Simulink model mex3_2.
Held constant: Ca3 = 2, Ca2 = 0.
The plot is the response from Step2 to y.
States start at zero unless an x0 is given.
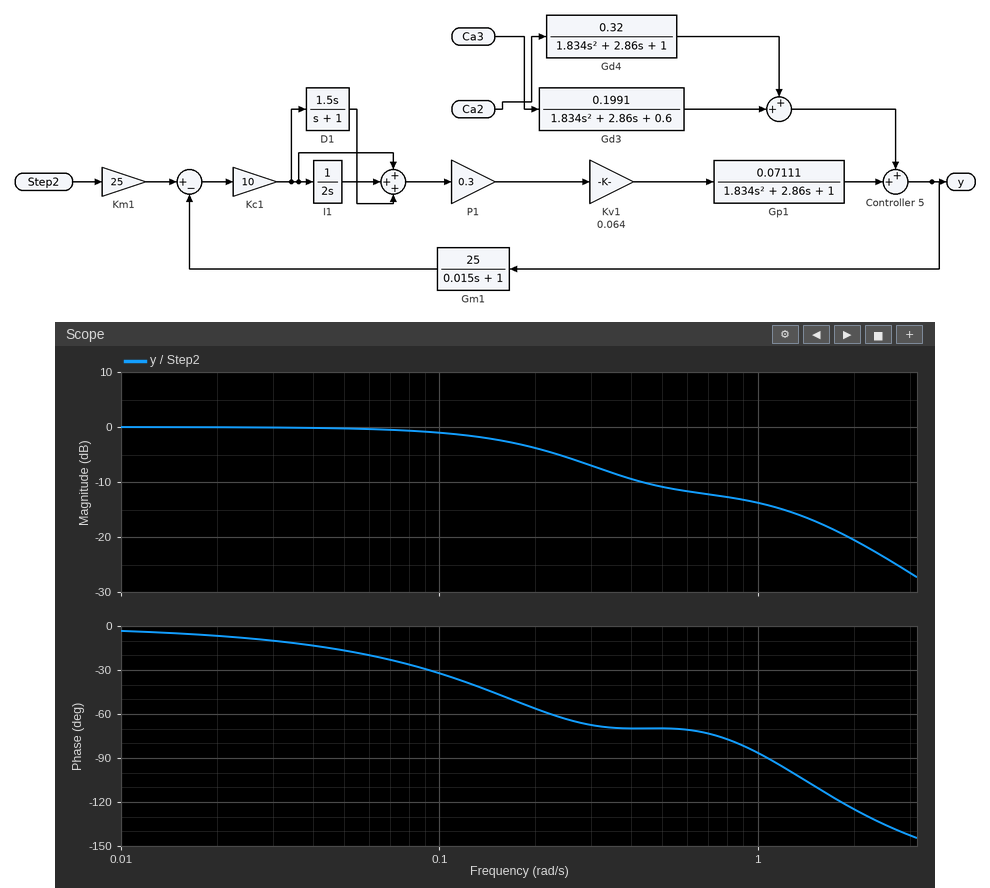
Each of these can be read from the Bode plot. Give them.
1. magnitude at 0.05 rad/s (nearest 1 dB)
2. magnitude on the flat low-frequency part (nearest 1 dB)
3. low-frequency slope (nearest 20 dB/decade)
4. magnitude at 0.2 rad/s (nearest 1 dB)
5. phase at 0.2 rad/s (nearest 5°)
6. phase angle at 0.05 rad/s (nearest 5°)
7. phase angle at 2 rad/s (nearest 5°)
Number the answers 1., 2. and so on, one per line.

1. 0 dB
2. 0 dB
3. 0 dB/decade
4. -4 dB
5. -55°
6. -15°
7. -125°
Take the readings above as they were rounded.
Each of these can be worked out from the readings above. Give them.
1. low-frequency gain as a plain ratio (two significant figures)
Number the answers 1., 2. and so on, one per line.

1. 1.0
